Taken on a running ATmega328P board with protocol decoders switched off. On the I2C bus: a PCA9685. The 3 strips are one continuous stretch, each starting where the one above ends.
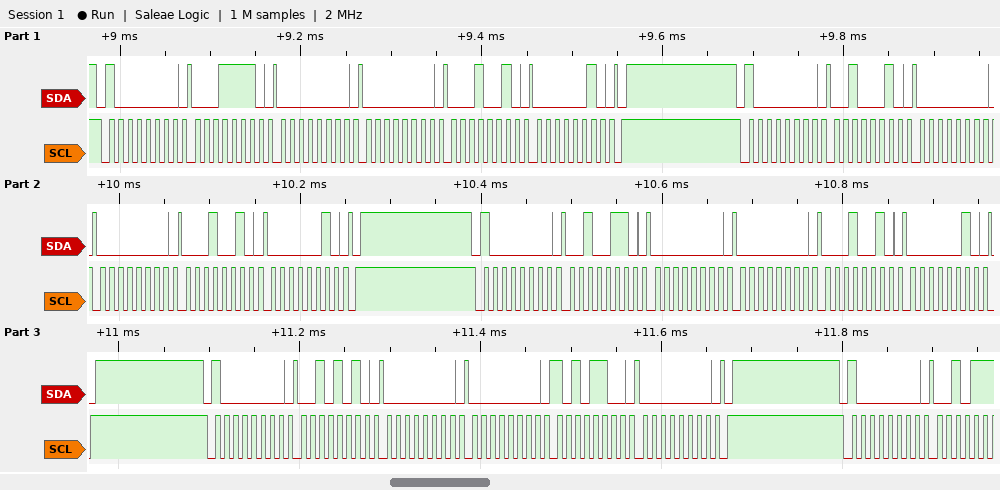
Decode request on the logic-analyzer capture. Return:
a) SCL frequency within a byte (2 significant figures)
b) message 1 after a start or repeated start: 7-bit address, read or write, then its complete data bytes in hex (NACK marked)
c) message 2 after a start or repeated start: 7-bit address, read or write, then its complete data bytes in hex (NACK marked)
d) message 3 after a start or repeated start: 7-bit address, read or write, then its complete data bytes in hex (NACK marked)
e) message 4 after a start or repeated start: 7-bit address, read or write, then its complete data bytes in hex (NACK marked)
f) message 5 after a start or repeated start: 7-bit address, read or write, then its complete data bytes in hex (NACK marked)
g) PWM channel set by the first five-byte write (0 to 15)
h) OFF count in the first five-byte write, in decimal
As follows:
100 kHz
0x40 write: 1E 00 00 12 02
0x40 write: 22 00 00 12 02
0x40 write: 26 00 00 12 02
0x40 write: 2A 00 00 AC 00
0x40 write
6
530
